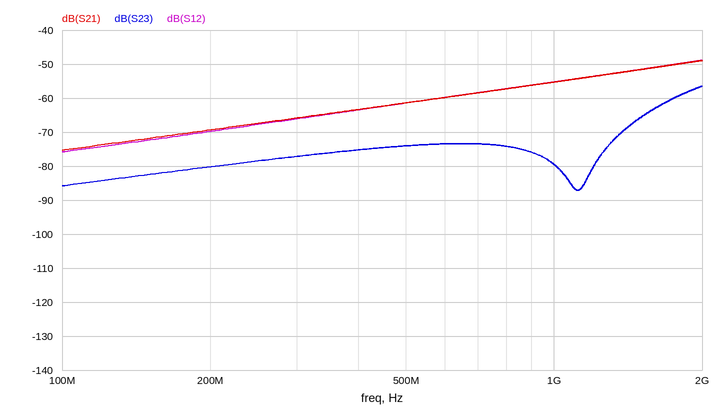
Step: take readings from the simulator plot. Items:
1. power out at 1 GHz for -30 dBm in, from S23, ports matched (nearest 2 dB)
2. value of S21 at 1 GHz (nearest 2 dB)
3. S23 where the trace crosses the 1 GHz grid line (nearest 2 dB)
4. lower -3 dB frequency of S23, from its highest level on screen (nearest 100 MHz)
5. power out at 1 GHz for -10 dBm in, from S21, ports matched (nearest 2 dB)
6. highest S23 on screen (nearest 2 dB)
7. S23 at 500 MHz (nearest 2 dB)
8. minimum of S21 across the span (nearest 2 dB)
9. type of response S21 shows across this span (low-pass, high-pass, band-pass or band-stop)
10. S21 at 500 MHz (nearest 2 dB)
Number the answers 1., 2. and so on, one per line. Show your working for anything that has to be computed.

1. -30 dBm + (-80 dB) = -110 dBm
2. -56 dB
3. -80 dB
4. 1.8 GHz
5. -10 dBm + (-56 dB) = -66 dBm
6. -56 dB
7. -74 dB
8. -76 dB
9. high-pass
10. -62 dB
